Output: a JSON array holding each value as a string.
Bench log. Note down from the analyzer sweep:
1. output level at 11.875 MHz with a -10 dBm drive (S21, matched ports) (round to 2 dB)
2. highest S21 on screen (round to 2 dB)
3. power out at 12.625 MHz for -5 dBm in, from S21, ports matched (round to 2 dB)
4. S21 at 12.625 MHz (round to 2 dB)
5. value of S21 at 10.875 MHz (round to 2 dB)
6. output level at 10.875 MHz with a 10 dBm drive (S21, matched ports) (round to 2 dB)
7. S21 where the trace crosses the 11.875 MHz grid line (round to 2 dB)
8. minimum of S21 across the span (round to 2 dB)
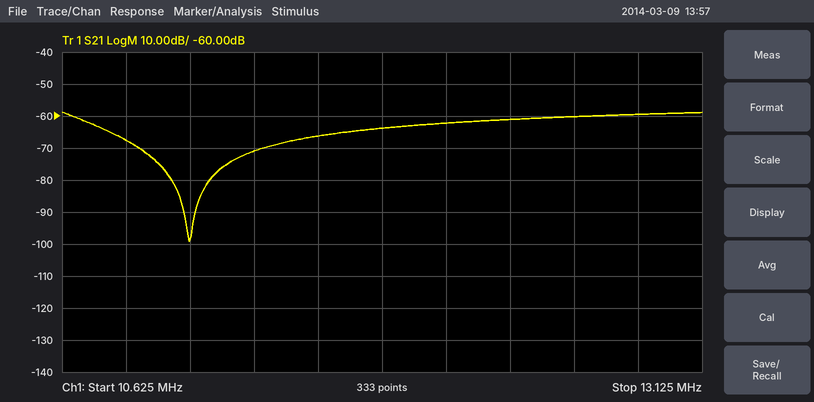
["-74 dBm", "-58 dB", "-66 dBm", "-60 dB", "-68 dB", "-58 dBm", "-64 dB", "-100 dB"]
